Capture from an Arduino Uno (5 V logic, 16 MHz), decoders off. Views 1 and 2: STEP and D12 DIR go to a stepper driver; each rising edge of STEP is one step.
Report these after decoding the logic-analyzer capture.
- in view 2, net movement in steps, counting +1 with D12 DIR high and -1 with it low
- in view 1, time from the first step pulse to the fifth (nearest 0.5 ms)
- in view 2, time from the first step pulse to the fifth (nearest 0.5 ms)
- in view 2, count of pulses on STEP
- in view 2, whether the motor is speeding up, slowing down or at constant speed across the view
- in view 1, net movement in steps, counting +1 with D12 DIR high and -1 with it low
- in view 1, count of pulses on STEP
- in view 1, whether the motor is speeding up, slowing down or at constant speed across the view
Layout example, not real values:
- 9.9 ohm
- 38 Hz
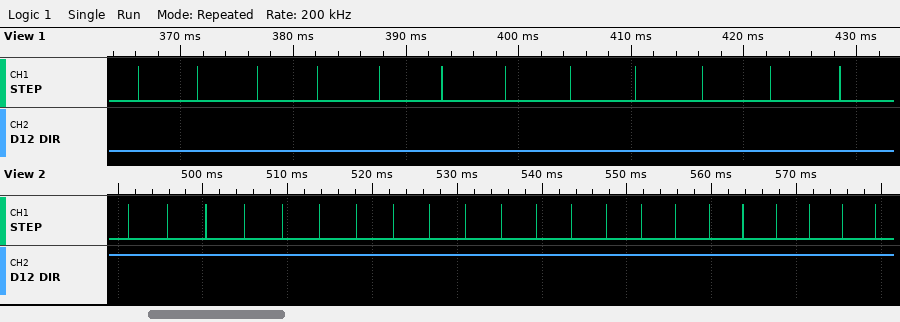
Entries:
- +22
- 21.5 ms
- 18.0 ms
- 22
- speeding up
- -12
- 12
- slowing down
